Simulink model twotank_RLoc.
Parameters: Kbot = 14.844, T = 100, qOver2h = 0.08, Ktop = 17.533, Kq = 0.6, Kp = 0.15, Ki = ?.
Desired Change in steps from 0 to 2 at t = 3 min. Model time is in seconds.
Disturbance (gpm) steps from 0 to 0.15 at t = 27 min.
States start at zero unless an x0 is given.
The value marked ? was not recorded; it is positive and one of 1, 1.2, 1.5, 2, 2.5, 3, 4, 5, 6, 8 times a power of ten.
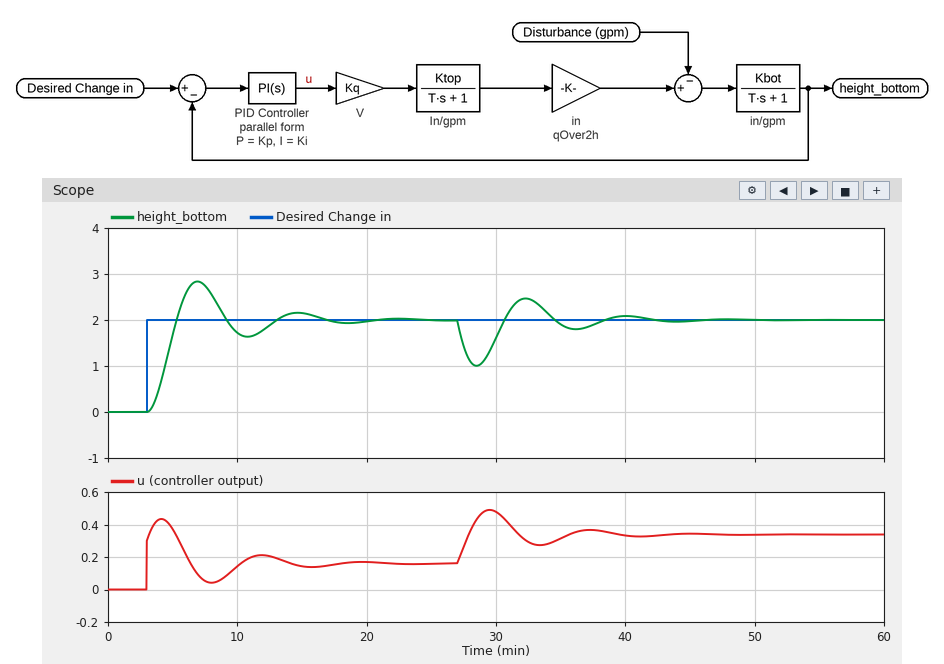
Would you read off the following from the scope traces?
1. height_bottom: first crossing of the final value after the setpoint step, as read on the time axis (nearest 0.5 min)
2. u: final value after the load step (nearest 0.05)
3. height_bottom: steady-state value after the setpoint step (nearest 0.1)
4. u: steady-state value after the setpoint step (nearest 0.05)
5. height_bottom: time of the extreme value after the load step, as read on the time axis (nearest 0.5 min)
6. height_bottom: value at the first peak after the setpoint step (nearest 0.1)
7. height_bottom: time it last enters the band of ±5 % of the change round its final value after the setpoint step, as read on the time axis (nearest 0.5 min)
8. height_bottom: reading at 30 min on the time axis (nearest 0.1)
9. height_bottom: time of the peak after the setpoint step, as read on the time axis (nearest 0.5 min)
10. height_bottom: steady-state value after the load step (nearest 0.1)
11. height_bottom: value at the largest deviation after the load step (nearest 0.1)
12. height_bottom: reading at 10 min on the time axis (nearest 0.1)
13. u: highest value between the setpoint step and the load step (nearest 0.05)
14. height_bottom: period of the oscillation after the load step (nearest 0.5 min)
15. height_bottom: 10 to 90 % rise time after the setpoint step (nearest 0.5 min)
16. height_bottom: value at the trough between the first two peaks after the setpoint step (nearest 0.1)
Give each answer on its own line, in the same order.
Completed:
5.5 min
0.35
2.0
0.15
28.5 min
2.8
16.0 min
1.6
7.0 min
2.0
1.0
1.7
0.45
7.5 min
1.5 min
1.6
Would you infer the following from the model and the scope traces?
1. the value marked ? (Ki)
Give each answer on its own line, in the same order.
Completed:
0.002
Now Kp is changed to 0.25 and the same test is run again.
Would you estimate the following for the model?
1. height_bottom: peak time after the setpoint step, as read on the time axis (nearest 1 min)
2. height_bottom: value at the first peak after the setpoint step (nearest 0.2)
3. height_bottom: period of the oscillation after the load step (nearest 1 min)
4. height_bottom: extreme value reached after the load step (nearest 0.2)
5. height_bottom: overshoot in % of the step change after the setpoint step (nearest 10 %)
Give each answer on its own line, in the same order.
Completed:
6 min
2.6
6 min
1.2
30 %
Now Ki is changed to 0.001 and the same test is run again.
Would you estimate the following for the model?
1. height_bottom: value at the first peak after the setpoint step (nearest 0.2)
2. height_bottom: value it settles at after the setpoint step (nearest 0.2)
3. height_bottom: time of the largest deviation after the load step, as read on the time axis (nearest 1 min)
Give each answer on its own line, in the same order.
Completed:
2.2
2.0
29 min
